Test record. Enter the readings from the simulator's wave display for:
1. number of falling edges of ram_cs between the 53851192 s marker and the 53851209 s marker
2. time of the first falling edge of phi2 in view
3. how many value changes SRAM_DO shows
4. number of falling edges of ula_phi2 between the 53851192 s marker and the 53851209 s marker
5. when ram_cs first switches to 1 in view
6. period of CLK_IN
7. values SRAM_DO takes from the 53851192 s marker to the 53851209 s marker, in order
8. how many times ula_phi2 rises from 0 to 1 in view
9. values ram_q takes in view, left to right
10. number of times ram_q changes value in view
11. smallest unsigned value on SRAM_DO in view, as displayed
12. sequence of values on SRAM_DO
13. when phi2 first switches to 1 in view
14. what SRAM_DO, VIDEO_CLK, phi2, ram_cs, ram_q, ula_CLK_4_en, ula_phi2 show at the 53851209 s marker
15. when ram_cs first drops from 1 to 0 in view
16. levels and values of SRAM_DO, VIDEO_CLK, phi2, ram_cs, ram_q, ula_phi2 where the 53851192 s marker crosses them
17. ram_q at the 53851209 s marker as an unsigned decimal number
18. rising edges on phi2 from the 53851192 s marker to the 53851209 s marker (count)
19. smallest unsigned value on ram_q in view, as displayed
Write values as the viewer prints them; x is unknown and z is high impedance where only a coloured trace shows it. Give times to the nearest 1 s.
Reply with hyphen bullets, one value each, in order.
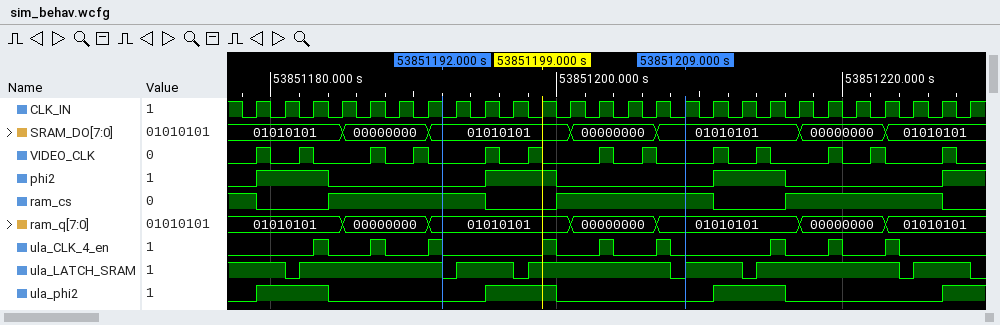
- 1
- 53851184 s
- 6
- 1
- 53851184 s
- 2 s
- 01010101, 00000000, 01010101
- 4
- 01010101, 00000000, 01010101, 00000000, 01010101, 00000000, 01010101
- 6
- 00000000
- 01010101, 00000000, 01010101, 00000000, 01010101, 00000000, 01010101
- 53851179 s
- SRAM_DO=01010101, VIDEO_CLK=0, phi2=0, ram_cs=1, ram_q=01010101, ula_CLK_4_en=0, ula_phi2=0
- 53851179 s
- SRAM_DO=01010101, VIDEO_CLK=0, phi2=0, ram_cs=1, ram_q=01010101, ula_phi2=0
- 85
- 1
- 00000000
